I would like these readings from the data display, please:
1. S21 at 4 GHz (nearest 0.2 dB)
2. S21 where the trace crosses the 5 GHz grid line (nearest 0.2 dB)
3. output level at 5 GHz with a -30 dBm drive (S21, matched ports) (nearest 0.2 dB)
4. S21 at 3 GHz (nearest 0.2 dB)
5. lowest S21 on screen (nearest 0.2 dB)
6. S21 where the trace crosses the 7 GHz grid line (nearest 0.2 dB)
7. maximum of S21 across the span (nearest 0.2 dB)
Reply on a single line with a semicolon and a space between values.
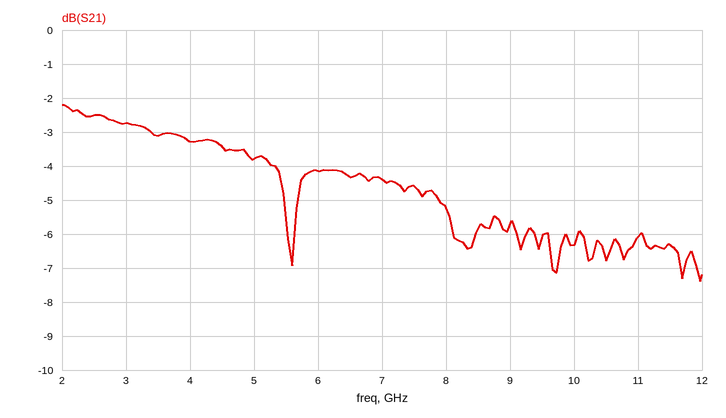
-3.2 dB; -3.8 dB; -33.8 dBm; -2.8 dB; -7.4 dB; -4.4 dB; -2.2 dB
